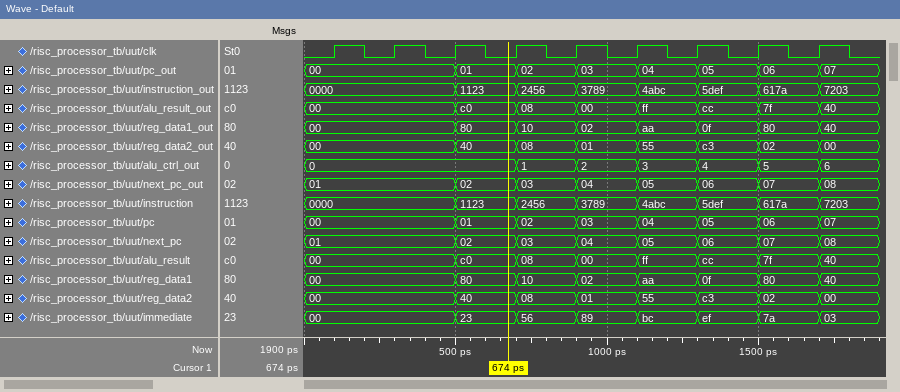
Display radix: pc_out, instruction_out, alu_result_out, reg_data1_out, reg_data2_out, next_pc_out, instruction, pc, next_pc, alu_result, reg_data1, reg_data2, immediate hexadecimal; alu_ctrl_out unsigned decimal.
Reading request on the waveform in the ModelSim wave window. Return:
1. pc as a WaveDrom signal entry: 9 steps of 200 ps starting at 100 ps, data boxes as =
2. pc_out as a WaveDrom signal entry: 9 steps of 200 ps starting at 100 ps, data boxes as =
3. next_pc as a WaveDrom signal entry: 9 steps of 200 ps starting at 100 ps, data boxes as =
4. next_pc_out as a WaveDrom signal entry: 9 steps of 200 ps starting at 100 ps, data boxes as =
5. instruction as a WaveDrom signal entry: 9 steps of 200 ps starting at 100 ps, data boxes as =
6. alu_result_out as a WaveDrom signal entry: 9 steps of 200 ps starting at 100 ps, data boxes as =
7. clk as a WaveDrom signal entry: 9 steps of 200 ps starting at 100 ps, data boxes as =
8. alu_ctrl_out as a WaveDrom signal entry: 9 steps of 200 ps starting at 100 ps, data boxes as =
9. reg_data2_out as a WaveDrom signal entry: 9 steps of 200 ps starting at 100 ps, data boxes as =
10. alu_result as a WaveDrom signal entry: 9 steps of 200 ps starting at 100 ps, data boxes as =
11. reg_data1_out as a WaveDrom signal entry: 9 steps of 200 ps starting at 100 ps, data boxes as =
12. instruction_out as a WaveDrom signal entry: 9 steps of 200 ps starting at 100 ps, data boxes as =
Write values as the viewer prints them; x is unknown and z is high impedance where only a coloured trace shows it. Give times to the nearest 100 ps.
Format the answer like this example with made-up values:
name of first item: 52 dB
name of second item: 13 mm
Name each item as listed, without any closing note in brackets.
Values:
pc as a WaveDrom signal entry: 9 steps of 200 ps starting at 100 ps, data boxes as =: {name: 'pc', wave: '=.=======', data: '00 01 02 03 04 05 06 07'}
pc_out as a WaveDrom signal entry: 9 steps of 200 ps starting at 100 ps, data boxes as =: {name: 'pc_out', wave: '=.=======', data: '00 01 02 03 04 05 06 07'}
next_pc as a WaveDrom signal entry: 9 steps of 200 ps starting at 100 ps, data boxes as =: {name: 'next_pc', wave: '=.=======', data: '01 02 03 04 05 06 07 08'}
next_pc_out as a WaveDrom signal entry: 9 steps of 200 ps starting at 100 ps, data boxes as =: {name: 'next_pc_out', wave: '=.=======', data: '01 02 03 04 05 06 07 08'}
instruction as a WaveDrom signal entry: 9 steps of 200 ps starting at 100 ps, data boxes as =: {name: 'instruction', wave: '=.=======', data: '0000 1123 2456 3789 4abc 5def 617a 7203'}
alu_result_out as a WaveDrom signal entry: 9 steps of 200 ps starting at 100 ps, data boxes as =: {name: 'alu_result_out', wave: '=.=======', data: '00 c0 08 00 ff cc 7f 40'}
clk as a WaveDrom signal entry: 9 steps of 200 ps starting at 100 ps, data boxes as =: {name: 'clk', wave: 'p........'}
alu_ctrl_out as a WaveDrom signal entry: 9 steps of 200 ps starting at 100 ps, data boxes as =: {name: 'alu_ctrl_out', wave: '=..======', data: '0 1 2 3 4 5 6'}
reg_data2_out as a WaveDrom signal entry: 9 steps of 200 ps starting at 100 ps, data boxes as =: {name: 'reg_data2_out', wave: '=.=======', data: '00 40 08 01 55 c3 02 00'}
alu_result as a WaveDrom signal entry: 9 steps of 200 ps starting at 100 ps, data boxes as =: {name: 'alu_result', wave: '=.=======', data: '00 c0 08 00 ff cc 7f 40'}
reg_data1_out as a WaveDrom signal entry: 9 steps of 200 ps starting at 100 ps, data boxes as =: {name: 'reg_data1_out', wave: '=.=======', data: '00 80 10 02 aa 0f 80 40'}
instruction_out as a WaveDrom signal entry: 9 steps of 200 ps starting at 100 ps, data boxes as =: {name: 'instruction_out', wave: '=.=======', data: '0000 1123 2456 3789 4abc 5def 617a 7203'}
